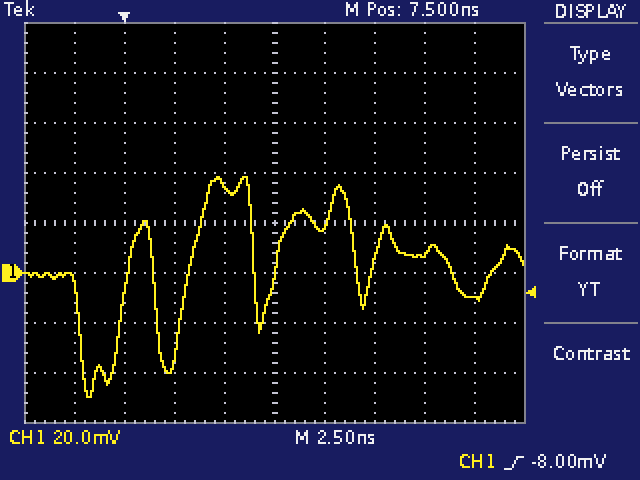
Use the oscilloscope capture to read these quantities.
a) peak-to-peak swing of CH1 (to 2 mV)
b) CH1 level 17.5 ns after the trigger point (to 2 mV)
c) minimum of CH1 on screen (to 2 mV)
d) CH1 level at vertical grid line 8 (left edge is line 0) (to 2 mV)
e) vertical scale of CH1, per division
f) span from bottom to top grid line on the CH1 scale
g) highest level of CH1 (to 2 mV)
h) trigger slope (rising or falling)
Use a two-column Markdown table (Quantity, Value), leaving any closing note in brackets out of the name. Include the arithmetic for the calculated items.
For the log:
| Quantity | Value |
|---|---|
| peak-to-peak swing of CH1 | 38 mV − (-50 mV) = 88 mV |
| CH1 level 17.5 ns after the trigger point | -10 mV |
| minimum of CH1 on screen | -50 mV |
| CH1 level at vertical grid line 8 (left edge is line 0) | 8 mV |
| vertical scale of CH1, per division | 20 mV |
| span from bottom to top grid line on the CH1 scale | 160 mV |
| highest level of CH1 | 38 mV |
| trigger slope | rising |
